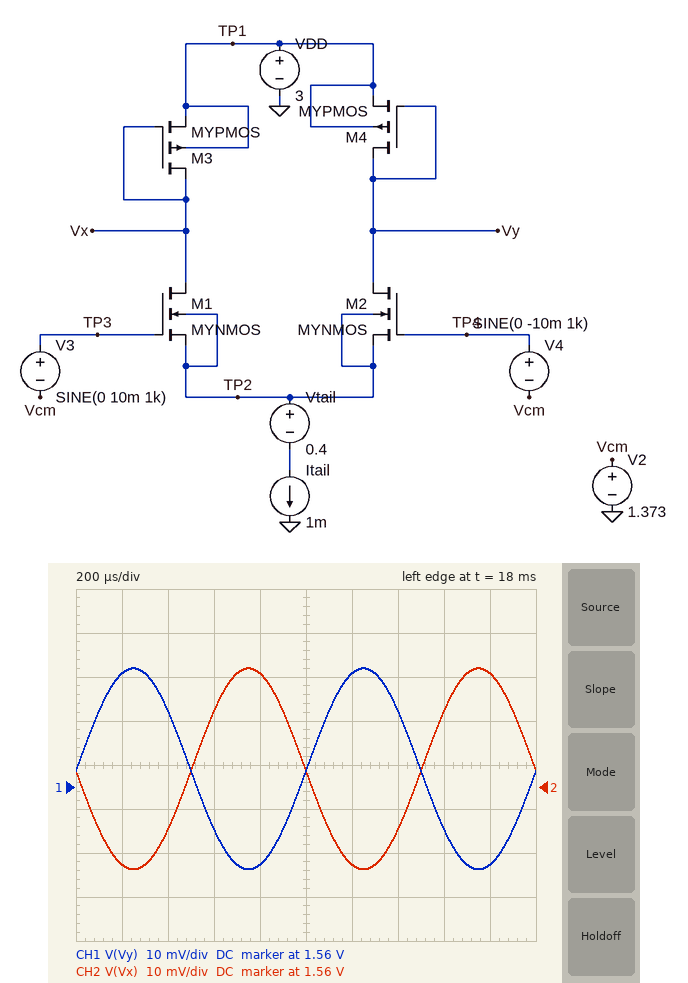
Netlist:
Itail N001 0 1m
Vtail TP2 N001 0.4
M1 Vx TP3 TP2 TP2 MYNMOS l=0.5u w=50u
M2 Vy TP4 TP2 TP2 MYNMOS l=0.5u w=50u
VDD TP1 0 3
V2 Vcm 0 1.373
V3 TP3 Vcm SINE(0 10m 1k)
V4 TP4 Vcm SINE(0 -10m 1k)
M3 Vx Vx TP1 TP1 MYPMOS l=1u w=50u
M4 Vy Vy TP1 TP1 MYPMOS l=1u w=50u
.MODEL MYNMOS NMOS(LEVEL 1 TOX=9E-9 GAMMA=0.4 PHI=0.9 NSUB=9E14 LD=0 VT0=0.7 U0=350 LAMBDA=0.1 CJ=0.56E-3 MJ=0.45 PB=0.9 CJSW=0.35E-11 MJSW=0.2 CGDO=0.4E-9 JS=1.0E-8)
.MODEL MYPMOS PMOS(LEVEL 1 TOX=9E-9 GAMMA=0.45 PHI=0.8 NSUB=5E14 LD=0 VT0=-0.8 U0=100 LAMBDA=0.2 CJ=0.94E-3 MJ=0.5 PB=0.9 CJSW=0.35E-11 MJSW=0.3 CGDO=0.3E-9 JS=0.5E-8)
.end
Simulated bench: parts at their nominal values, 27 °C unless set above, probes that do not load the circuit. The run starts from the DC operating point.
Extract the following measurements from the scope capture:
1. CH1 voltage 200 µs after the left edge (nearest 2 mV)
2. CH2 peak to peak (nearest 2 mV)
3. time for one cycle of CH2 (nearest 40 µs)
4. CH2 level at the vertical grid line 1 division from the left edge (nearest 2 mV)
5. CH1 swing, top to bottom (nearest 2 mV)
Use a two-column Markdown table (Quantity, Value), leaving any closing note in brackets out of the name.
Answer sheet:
| Quantity | Value |
|---|---|
| CH1 voltage 200 µs after the left edge | 1.586 V |
| CH2 peak to peak | 46 mV |
| time for one cycle of CH2 | 1.00 ms |
| CH2 level at the vertical grid line 1 division from the left edge | 1.542 V |
| CH1 swing, top to bottom | 46 mV |
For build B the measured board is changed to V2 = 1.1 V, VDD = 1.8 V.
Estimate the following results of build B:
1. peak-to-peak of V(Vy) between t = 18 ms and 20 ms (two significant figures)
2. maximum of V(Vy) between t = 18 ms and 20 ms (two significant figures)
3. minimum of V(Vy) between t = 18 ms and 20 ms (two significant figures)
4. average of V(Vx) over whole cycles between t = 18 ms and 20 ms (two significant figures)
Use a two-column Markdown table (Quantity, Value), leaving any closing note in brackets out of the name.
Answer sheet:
| Quantity | Value |
|---|---|
| peak-to-peak of V(Vy) between t = 18 ms and 20 ms | 30 mV |
| maximum of V(Vy) between t = 18 ms and 20 ms | 380 mV |
| minimum of V(Vy) between t = 18 ms and 20 ms | 350 mV |
| average of V(Vx) over whole cycles between t = 18 ms and 20 ms | 360 mV |
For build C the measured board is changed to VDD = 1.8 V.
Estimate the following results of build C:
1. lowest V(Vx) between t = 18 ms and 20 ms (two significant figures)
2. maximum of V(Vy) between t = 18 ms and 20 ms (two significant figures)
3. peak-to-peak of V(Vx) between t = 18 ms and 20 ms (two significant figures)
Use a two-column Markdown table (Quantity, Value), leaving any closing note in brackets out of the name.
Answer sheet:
| Quantity | Value |
|---|---|
| lowest V(Vx) between t = 18 ms and 20 ms | 360 mV |
| maximum of V(Vy) between t = 18 ms and 20 ms | 370 mV |
| peak-to-peak of V(Vx) between t = 18 ms and 20 ms | 4.7 mV |
